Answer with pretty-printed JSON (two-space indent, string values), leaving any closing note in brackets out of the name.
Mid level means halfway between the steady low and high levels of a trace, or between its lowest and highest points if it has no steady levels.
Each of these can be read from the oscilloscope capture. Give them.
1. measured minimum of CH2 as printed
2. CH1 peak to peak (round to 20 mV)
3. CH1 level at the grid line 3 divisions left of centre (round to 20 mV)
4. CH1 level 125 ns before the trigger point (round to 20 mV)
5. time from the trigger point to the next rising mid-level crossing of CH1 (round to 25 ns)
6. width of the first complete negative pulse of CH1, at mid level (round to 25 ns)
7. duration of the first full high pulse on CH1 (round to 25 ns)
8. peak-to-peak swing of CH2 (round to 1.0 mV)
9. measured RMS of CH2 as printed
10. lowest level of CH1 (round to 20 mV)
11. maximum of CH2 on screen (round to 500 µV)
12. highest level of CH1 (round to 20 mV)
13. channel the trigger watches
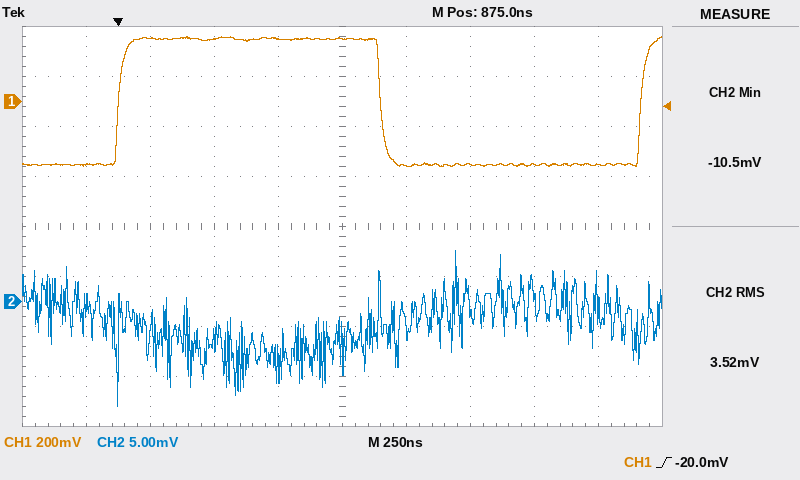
{
  "measured minimum of CH2 as printed": "-10.5 mV",
  "CH1 peak to peak": "520 mV",
  "CH1 level at the grid line 3 divisions left of centre": "260 mV",
  "CH1 level 125 ns before the trigger point": "-260 mV",
  "time from the trigger point to the next rising mid-level crossing of CH1": "2.050 µs",
  "width of the first complete negative pulse of CH1, at mid level": "1.025 µs",
  "duration of the first full high pulse on CH1": "1.025 µs",
  "peak-to-peak swing of CH2": "16.0 mV",
  "measured RMS of CH2 as printed": "3.52 mV",
  "lowest level of CH1": "-260 mV",
  "maximum of CH2 on screen": "5.0 mV",
  "highest level of CH1": "260 mV",
  "channel the trigger watches": "CH1"
}
